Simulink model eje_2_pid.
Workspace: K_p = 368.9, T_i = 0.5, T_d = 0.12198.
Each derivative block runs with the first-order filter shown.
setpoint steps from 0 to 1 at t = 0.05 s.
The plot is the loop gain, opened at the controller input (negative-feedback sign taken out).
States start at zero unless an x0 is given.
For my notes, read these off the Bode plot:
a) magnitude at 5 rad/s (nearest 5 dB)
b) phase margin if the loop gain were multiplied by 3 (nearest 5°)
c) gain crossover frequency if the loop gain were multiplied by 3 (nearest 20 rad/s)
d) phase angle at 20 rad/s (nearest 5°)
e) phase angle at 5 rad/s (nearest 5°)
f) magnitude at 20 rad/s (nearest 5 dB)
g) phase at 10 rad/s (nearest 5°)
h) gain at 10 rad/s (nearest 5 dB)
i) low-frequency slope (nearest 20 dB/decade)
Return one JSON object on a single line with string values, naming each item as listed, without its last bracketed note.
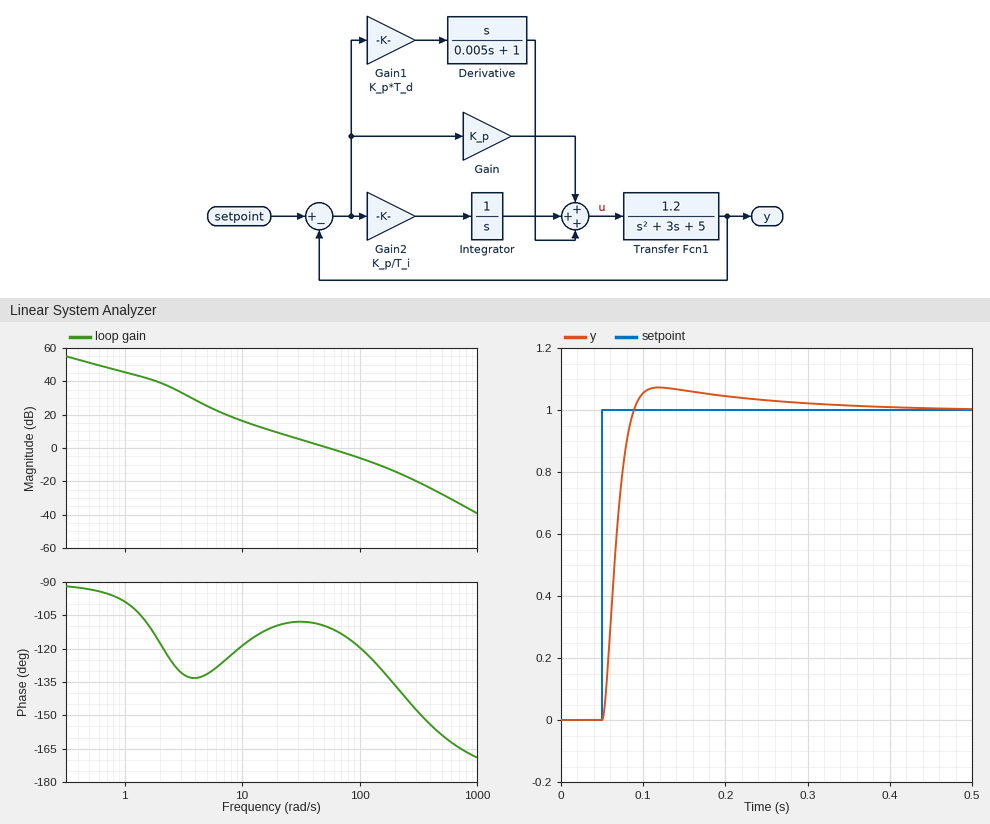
{"magnitude at 5 rad/s": "25 dB", "phase margin if the loop gain were multiplied by 3": "55°", "gain crossover frequency if the loop gain were multiplied by 3": "140 rad/s", "phase angle at 20 rad/s": "-110°", "phase angle at 5 rad/s": "-130°", "magnitude at 20 rad/s": "10 dB", "phase at 10 rad/s": "-120°", "gain at 10 rad/s": "15 dB", "low-frequency slope": "-20 dB/decade"}
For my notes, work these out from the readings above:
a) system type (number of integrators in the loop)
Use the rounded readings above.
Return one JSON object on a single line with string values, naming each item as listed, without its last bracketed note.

{"system type": "1"}
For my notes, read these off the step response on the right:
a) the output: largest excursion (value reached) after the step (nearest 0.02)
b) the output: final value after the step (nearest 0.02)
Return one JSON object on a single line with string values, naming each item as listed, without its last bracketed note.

{"the output: largest excursion (value reached) after the step": "1.08", "the output: final value after the step": "1.00"}
